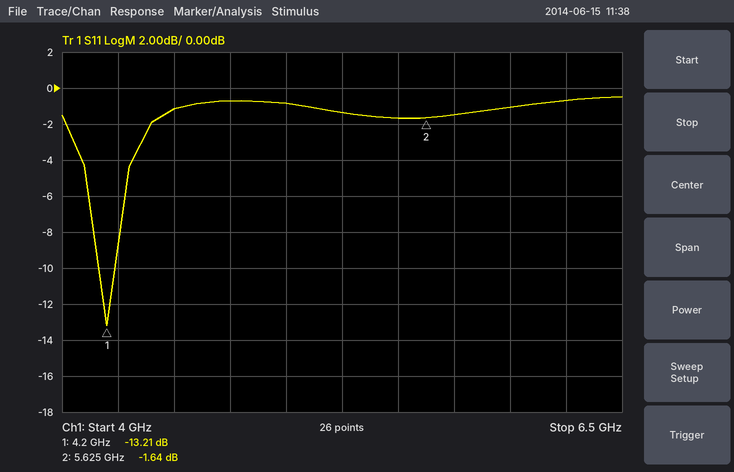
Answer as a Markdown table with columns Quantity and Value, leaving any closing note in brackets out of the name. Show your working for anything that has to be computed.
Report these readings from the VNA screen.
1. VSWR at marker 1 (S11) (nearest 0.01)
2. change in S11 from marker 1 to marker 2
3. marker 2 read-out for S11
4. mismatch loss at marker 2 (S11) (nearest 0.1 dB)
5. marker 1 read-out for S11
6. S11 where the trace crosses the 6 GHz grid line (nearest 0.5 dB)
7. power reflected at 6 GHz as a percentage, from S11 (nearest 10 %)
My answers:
| Quantity | Value |
|---|---|
| VSWR at marker 1 (S11) | (1 + 0.2185)/(1 − 0.2185) ≈ 1.56 |
| change in S11 from marker 1 to marker 2 | -1.64 − (-13.21) = 11.57 dB |
| marker 2 read-out for S11 | -1.64 dB |
| mismatch loss at marker 2 (S11) | −10 log10(1 − 10^(-1.64/10)) ≈ 5.0 dB |
| marker 1 read-out for S11 | -13.21 dB |
| S11 where the trace crosses the 6 GHz grid line | -1.0 dB |
| power reflected at 6 GHz as a percentage, from S11 | 10^(-1/10) ≈ 79.4 %, so 80 % to the nearest 10 % |
